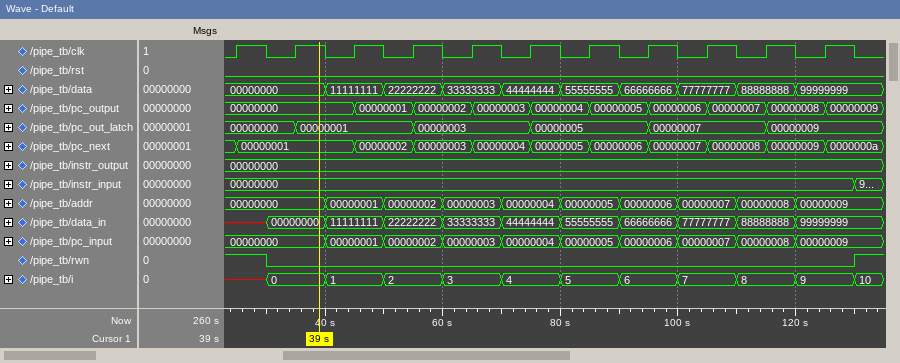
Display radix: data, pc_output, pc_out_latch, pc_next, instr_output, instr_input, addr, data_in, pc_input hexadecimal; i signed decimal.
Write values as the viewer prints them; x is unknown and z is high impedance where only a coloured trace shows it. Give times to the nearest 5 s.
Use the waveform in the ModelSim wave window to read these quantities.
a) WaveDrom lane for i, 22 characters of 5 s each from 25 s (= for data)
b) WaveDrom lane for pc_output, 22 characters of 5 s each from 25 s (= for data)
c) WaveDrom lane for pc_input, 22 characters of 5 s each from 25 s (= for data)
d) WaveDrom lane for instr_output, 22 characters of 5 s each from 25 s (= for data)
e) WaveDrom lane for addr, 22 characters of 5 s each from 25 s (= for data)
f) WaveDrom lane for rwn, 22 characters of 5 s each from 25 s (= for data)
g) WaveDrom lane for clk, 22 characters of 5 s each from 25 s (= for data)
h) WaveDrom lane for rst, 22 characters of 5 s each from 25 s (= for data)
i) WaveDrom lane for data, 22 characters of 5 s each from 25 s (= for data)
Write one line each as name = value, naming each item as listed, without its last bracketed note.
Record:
WaveDrom lane for i, 22 characters of 5 s each from 25 s = {name: 'i', wave: 'x=.=.=.=.=.=.=.=.=.=.=', data: '0 1 2 3 4 5 6 7 8 9 10'}
WaveDrom lane for pc_output, 22 characters of 5 s each from 25 s = {name: 'pc_output', wave: '=...=.=.=.=.=.=.=.=.=.', data: '00000000 00000001 00000002 00000003 00000004 00000005 00000006 00000007 00000008 00000009'}
WaveDrom lane for pc_input, 22 characters of 5 s each from 25 s = {name: 'pc_input', wave: '=..=.=.=.=.=.=.=.=.=..', data: '00000000 00000001 00000002 00000003 00000004 00000005 00000006 00000007 00000008 00000009'}
WaveDrom lane for instr_output, 22 characters of 5 s each from 25 s = {name: 'instr_output', wave: '=.....................', data: '00000000'}
WaveDrom lane for addr, 22 characters of 5 s each from 25 s = {name: 'addr', wave: '=..=.=.=.=.=.=.=.=.=..', data: '00000000 00000001 00000002 00000003 00000004 00000005 00000006 00000007 00000008 00000009'}
WaveDrom lane for rwn, 22 characters of 5 s each from 25 s = {name: 'rwn', wave: '10...................1'}
WaveDrom lane for clk, 22 characters of 5 s each from 25 s = {name: 'clk', wave: '1010101010101010101010'}
WaveDrom lane for rst, 22 characters of 5 s each from 25 s = {name: 'rst', wave: '0.....................'}
WaveDrom lane for data, 22 characters of 5 s each from 25 s = {name: 'data', wave: '=..=.=.=.=.=.=.=.=.=..', data: '00000000 11111111 22222222 33333333 44444444 55555555 66666666 77777777 88888888 99999999'}
